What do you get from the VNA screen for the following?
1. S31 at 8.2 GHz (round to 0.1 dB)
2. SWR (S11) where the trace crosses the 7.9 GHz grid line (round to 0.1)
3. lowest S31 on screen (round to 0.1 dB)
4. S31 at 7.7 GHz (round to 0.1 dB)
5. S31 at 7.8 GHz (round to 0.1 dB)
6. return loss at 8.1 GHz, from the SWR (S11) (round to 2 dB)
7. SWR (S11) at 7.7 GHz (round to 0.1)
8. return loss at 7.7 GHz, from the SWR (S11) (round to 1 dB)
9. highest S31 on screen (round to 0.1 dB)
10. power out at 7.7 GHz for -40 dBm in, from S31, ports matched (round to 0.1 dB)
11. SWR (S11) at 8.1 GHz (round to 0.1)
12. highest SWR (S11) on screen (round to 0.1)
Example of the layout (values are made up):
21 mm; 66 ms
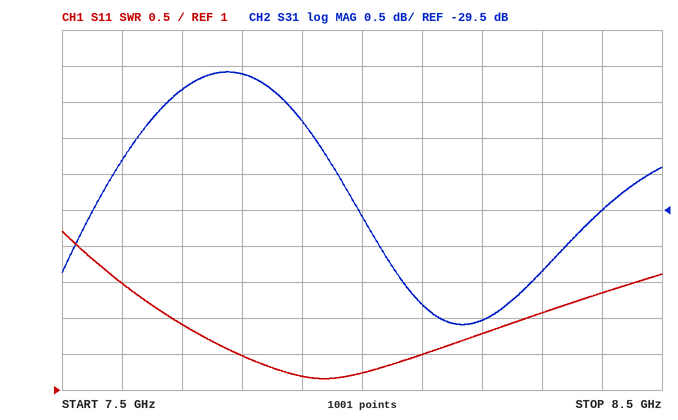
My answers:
-31.0 dB; 1.2; -31.1 dB; -27.8 dB; -27.6 dB; 14 dB; 1.9; 10 dB; -27.6 dB; -67.8 dBm; 1.5; 3.2
